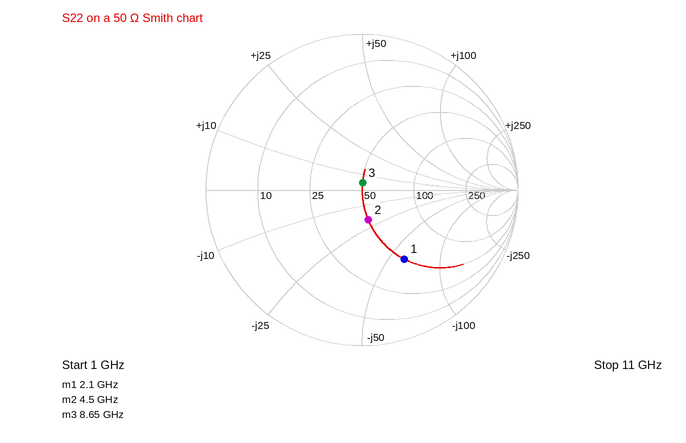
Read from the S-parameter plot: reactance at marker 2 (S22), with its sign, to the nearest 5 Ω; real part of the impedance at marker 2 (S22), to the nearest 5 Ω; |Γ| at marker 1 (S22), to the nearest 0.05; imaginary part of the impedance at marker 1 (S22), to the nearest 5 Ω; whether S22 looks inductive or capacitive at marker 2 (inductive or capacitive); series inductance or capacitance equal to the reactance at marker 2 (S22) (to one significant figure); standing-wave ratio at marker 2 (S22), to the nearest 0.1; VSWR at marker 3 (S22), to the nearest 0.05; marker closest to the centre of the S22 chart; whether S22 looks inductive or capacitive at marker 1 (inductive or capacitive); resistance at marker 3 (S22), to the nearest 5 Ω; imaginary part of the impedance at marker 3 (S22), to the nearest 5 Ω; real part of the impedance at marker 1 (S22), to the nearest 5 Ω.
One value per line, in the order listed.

-20 Ω
50 Ω
0.50
-60 Ω
capacitive
2 pF
1.5
1.10
marker 3
capacitive
50 Ω
+5 Ω
50 Ω
